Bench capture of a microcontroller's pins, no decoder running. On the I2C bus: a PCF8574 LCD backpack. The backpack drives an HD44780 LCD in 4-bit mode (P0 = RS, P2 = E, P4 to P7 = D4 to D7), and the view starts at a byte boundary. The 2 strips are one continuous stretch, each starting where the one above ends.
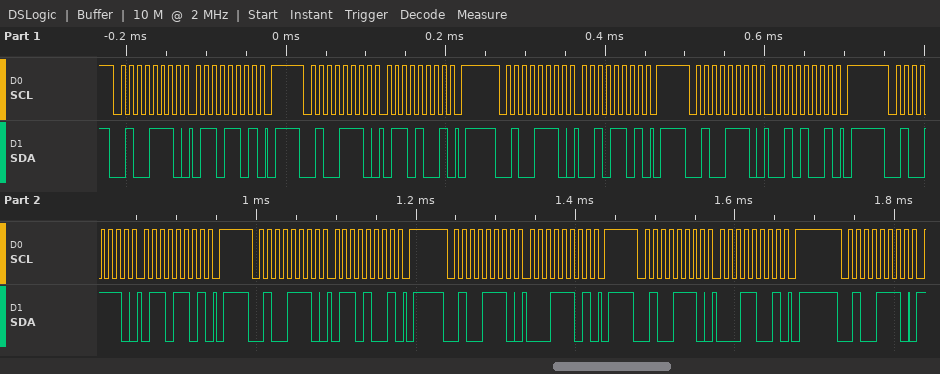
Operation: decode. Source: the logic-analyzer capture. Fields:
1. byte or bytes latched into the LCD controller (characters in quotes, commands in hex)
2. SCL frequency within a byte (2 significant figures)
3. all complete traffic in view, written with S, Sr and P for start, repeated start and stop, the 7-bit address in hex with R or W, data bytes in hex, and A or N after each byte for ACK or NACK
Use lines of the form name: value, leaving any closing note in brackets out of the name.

byte or bytes latched into the LCD controller: 'b' 'a'
SCL frequency within a byte: 100 kHz
all complete traffic in view, written with S, Sr and P for start, repeated start and stop, the 7-bit address in hex with R or W, data bytes in hex, and A or N after each byte for ACK or NACK: S 27W A 6D A P S 27W A 69 A P S 27W A 2D A P S 27W A 29 A P S 27W A 6D A P S 27W A 69 A P S 27W A 1D A P S 27W A 19 A P S 27W A
